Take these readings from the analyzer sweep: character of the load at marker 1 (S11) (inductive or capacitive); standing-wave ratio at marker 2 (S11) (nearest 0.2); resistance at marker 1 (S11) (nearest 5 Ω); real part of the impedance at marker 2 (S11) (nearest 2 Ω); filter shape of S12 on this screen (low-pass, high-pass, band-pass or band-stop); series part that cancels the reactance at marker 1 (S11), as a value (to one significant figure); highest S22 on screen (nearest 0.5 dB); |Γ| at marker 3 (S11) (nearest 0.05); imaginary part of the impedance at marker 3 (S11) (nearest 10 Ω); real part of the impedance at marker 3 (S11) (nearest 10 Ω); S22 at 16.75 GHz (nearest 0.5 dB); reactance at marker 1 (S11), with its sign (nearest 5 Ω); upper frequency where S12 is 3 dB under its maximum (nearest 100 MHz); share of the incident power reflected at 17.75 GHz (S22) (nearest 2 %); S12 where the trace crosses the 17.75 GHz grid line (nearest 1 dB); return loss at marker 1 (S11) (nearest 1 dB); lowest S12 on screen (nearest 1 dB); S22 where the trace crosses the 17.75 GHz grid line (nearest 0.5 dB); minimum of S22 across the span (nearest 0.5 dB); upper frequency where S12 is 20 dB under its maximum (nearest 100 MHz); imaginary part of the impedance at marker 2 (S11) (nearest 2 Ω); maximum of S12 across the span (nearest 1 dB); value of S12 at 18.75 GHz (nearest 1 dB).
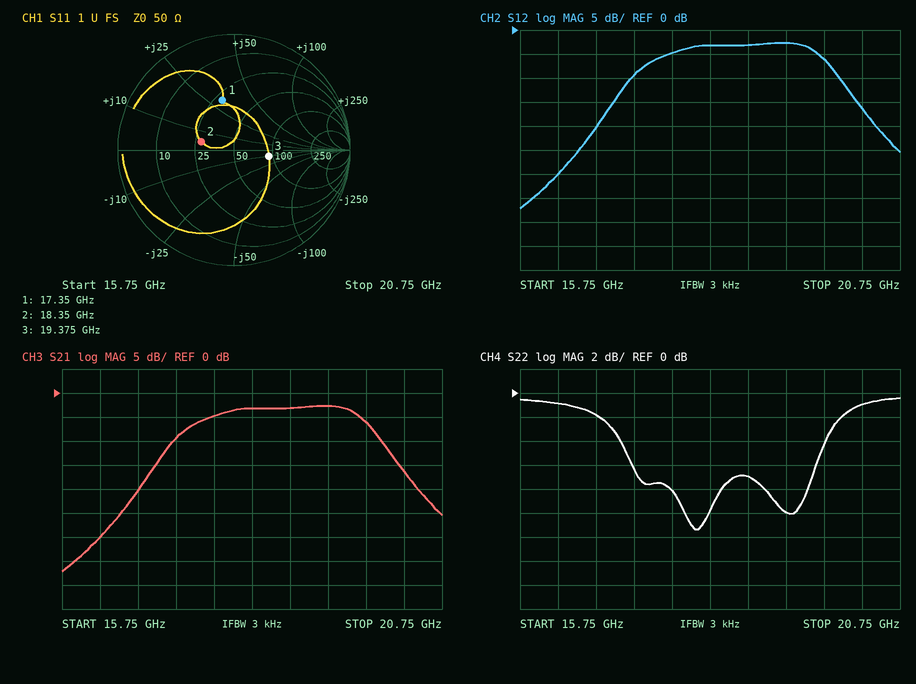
inductive
1.8
30 Ω
28 Ω
band-pass
300 fF
-0.5 dB
0.30
-10 Ω
90 Ω
-2.0 dB
+30 Ω
19.7 GHz
16 %
-5 dB
7 dB
-37 dB
-8.0 dB
-11.5 dB
20.6 GHz
+4 Ω
-3 dB
-3 dB
